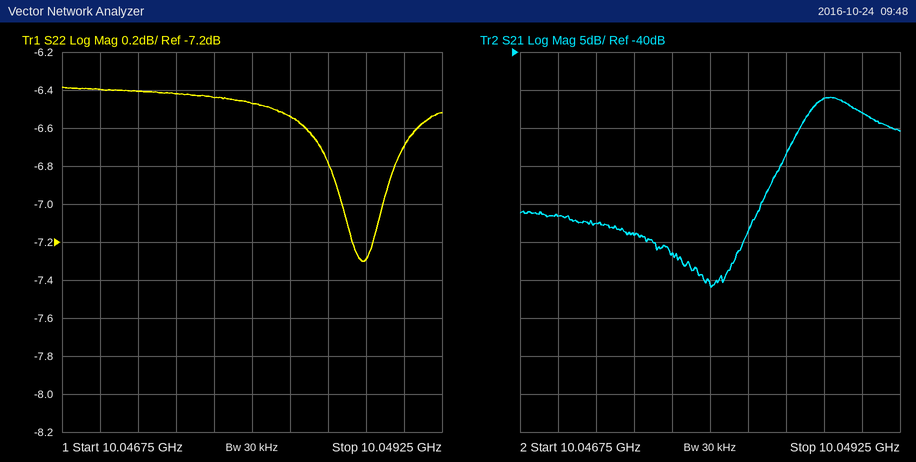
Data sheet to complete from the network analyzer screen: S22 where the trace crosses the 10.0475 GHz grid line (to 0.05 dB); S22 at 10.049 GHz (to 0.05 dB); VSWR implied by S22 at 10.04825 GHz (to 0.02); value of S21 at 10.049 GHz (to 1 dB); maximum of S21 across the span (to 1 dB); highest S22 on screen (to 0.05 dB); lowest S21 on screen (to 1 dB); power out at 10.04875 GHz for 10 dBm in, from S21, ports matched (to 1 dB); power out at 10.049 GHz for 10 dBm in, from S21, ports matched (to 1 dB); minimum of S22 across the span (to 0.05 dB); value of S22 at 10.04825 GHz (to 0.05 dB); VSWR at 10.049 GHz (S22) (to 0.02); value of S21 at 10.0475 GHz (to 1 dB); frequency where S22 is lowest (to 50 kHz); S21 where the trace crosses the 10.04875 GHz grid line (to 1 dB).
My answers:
-6.40 dB
-6.70 dB
2.78
-48 dB
-46 dB
-6.40 dB
-71 dB
-36 dBm
-38 dBm
-7.30 dB
-6.55 dB
2.72
-64 dB
10.04875 GHz
-46 dB
